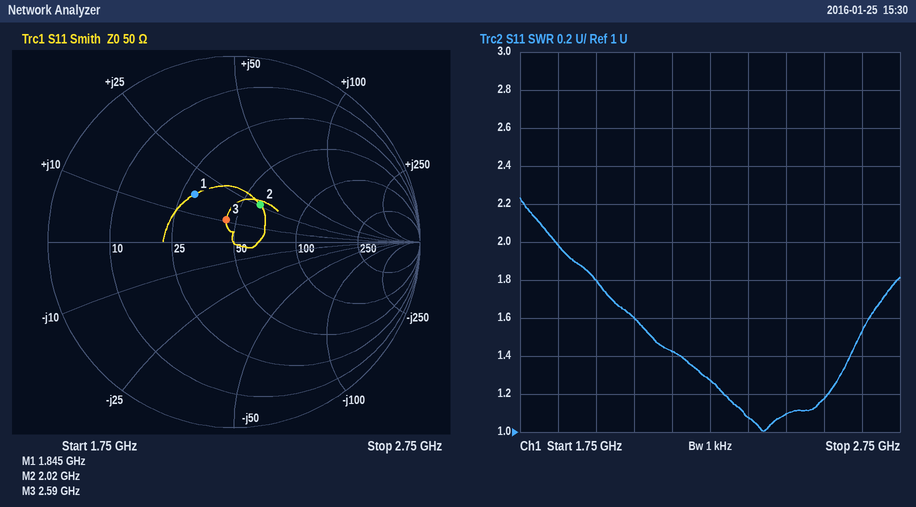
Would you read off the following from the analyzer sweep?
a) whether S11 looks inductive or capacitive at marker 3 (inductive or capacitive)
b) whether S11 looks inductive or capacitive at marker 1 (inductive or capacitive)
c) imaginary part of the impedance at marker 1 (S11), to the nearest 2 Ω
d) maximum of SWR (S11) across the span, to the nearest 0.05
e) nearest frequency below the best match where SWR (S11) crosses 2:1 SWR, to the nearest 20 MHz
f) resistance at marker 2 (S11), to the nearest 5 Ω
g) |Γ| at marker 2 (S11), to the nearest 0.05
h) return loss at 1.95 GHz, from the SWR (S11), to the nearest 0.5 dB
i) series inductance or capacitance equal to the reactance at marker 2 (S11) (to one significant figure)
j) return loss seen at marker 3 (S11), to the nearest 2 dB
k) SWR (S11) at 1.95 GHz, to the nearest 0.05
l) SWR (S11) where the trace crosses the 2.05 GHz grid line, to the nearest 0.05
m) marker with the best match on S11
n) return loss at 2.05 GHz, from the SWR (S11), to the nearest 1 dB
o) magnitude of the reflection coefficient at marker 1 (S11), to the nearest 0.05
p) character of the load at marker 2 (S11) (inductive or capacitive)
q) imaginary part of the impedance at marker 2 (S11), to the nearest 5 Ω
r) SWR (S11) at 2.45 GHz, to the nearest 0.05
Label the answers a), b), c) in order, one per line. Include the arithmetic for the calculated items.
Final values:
a) inductive
b) inductive
c) +16 Ω
d) 2.25
e) 1.84 GHz
f) 60 Ω
g) 0.25
h) −20 log10((1.8 − 1)/(1.8 + 1)) ≈ 10.9 dB, so 11.0 dB to the nearest 0.5 dB
i) L = 25 Ω/(2π × 2.02 GHz) ≈ 2 nH
j) 18 dB
k) 1.80
l) 1.60
m) marker 3
n) −20 log10((1.6 − 1)/(1.6 + 1)) ≈ 13 dB
o) 0.35
p) inductive
q) +25 Ω
r) 1.10
